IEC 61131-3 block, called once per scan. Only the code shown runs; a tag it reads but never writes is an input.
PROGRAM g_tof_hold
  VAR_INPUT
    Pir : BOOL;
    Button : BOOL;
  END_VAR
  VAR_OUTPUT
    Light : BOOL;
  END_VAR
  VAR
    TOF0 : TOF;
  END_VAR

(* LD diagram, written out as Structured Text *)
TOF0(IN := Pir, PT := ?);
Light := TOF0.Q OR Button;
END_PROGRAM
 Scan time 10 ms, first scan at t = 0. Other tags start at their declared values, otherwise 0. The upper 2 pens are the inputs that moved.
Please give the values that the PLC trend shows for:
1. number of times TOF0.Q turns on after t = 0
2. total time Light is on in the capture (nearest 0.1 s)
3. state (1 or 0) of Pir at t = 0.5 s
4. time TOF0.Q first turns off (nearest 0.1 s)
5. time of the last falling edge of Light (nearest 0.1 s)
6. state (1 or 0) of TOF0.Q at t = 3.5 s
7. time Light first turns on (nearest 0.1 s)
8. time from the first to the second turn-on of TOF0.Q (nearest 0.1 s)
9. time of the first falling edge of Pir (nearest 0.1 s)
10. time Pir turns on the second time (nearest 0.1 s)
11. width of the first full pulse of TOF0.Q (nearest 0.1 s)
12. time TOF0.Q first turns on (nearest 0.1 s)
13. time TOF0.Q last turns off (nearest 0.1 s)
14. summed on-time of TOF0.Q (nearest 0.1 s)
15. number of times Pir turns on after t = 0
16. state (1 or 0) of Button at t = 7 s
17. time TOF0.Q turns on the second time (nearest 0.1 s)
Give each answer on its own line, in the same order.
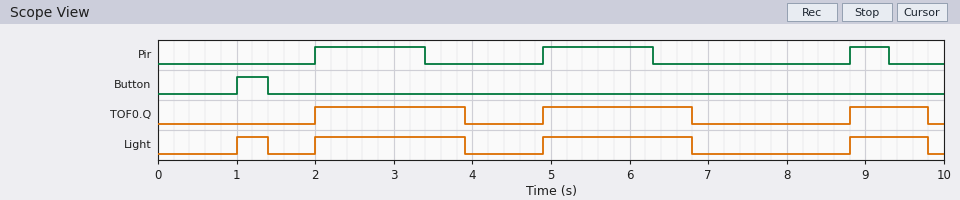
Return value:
3
5.2 s
0
3.9 s
9.8 s
1
1.0 s
2.9 s
3.4 s
4.9 s
1.9 s
2.0 s
9.8 s
4.8 s
3
0
4.9 s
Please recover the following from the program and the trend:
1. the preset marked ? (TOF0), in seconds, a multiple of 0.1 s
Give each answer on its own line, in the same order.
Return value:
0.5 s
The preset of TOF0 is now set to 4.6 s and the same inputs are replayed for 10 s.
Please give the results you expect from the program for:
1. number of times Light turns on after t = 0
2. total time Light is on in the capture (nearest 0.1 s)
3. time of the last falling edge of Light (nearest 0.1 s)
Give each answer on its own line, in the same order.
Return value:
2
8.4 s
1.4 s
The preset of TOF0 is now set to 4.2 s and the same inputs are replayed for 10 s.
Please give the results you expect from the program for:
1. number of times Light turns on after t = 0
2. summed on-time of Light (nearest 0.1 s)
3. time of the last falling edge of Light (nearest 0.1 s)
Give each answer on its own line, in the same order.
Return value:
2
8.4 s
1.4 s
